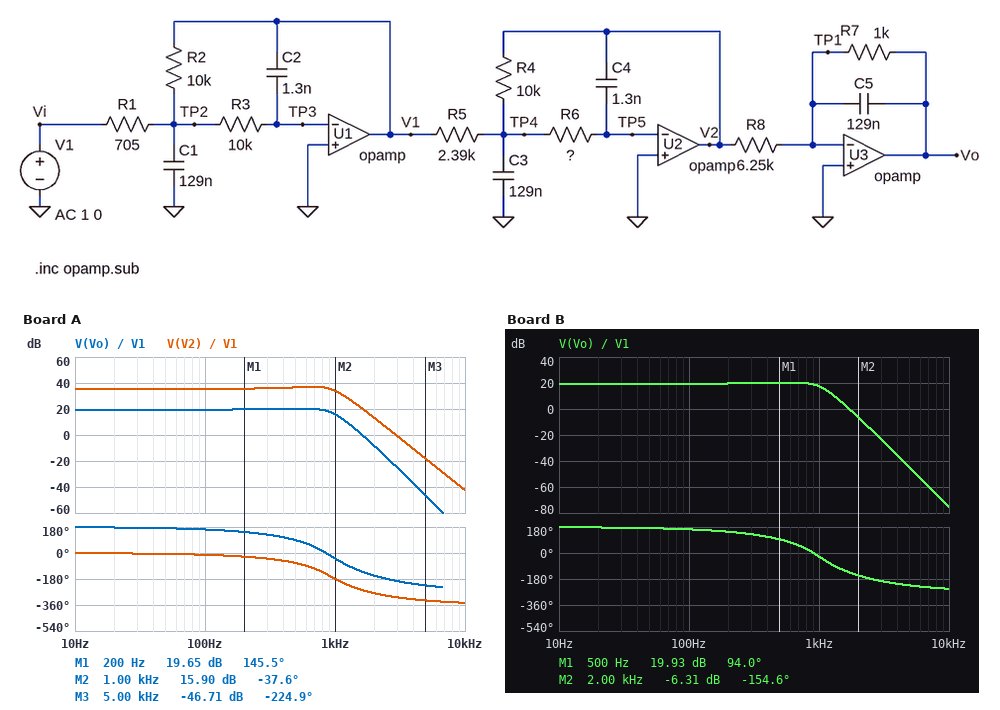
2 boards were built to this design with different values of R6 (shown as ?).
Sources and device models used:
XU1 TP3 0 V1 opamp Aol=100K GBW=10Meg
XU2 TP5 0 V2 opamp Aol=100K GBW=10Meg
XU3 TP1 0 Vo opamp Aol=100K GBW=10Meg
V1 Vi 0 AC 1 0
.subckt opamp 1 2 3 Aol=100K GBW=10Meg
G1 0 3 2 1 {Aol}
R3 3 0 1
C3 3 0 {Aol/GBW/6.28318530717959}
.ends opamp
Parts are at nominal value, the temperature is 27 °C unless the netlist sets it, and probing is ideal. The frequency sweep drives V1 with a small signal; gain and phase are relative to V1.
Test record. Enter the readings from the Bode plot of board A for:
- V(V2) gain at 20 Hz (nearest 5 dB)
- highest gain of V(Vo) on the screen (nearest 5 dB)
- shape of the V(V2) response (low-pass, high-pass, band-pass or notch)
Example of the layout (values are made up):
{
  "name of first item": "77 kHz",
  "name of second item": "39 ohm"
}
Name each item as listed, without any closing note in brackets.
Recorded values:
{
  "V(V2) gain at 20 Hz": "35 dB",
  "highest gain of V(Vo) on the screen": "20 dB",
  "shape of the V(V2) response": "low-pass"
}
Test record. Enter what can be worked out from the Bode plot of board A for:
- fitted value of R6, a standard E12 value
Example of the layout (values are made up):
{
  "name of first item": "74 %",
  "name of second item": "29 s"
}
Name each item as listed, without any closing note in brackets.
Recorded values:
{
  "fitted value of R6, a standard E12 value": "18 kΩ"
}
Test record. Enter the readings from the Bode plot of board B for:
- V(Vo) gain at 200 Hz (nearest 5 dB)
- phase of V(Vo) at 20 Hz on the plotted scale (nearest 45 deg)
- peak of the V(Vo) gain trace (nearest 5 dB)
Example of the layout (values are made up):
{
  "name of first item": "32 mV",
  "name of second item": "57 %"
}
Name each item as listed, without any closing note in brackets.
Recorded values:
{
  "V(Vo) gain at 200 Hz": "20 dB",
  "phase of V(Vo) at 20 Hz on the plotted scale": "180 deg",
  "peak of the V(Vo) gain trace": "20 dB"
}
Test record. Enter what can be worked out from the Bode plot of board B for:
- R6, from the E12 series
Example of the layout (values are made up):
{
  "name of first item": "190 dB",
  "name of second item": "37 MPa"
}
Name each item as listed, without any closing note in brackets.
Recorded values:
{
  "R6, from the E12 series": "15 kΩ"
}
